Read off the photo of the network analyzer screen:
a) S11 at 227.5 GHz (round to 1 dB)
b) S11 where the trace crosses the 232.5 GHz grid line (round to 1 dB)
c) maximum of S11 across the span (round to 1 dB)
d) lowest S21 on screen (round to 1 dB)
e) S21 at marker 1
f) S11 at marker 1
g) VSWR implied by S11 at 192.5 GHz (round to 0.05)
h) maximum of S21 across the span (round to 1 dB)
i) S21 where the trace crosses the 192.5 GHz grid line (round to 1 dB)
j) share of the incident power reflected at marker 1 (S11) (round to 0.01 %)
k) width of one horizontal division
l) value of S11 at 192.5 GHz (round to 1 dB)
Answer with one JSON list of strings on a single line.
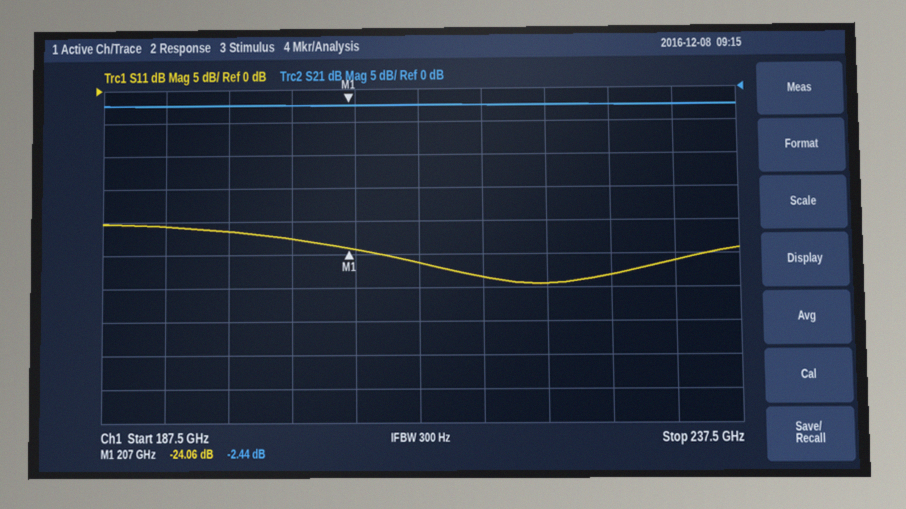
["-28 dB", "-26 dB", "-20 dB", "-3 dB", "-2.44 dB", "-24.06 dB", "1.20", "-2 dB", "-2 dB", "0.39 %", "5 GHz", "-21 dB"]
